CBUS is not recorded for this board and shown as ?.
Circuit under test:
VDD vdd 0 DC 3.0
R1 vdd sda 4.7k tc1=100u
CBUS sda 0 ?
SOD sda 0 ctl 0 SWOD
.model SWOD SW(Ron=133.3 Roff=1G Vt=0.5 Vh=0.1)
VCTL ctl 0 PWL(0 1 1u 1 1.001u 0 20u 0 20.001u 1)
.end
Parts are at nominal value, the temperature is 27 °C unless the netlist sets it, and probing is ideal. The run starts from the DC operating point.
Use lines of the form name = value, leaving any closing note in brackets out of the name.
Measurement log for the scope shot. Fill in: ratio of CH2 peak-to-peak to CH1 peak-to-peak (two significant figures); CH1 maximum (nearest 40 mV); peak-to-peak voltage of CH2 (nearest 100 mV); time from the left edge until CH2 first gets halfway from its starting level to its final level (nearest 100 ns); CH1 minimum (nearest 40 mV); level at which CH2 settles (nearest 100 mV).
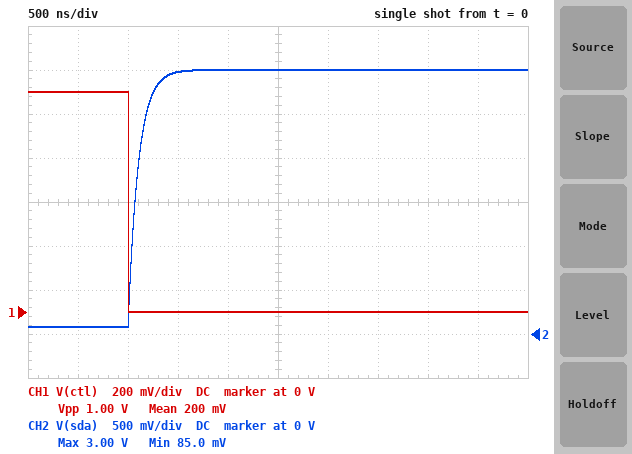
ratio of CH2 peak-to-peak to CH1 peak-to-peak = 2.9
CH1 maximum = 1.00 V
peak-to-peak voltage of CH2 = 2.9 V
time from the left edge until CH2 first gets halfway from its starting level to its final level = 1.1 µs
CH1 minimum = 0 V
level at which CH2 settles = 3.0 V
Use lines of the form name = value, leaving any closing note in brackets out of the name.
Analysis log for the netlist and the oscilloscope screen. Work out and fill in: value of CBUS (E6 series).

value of CBUS = 22 pF
